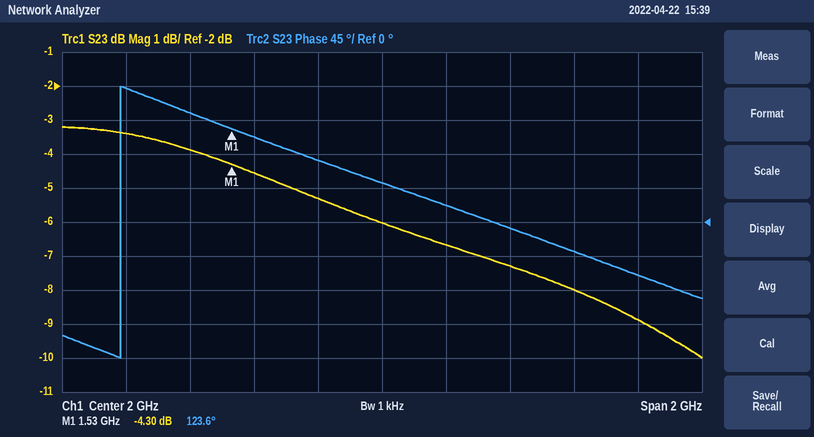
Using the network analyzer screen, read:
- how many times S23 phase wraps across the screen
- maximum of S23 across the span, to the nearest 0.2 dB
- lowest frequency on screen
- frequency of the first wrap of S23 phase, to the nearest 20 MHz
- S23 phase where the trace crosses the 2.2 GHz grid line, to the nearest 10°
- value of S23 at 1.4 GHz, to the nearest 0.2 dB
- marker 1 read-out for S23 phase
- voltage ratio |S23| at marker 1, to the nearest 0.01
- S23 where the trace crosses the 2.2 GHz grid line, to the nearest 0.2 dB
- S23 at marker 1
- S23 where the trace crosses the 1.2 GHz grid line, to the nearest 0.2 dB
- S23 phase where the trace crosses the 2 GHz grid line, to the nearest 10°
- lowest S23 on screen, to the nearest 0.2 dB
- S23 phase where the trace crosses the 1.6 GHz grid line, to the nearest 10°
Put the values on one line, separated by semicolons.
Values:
1; -3.2 dB; 1 GHz; 1.18 GHz; 20°; -3.8 dB; 123.6°; 0.61; -6.6 dB; -4.30 dB; -3.4 dB; 50°; -10.0 dB; 110°
